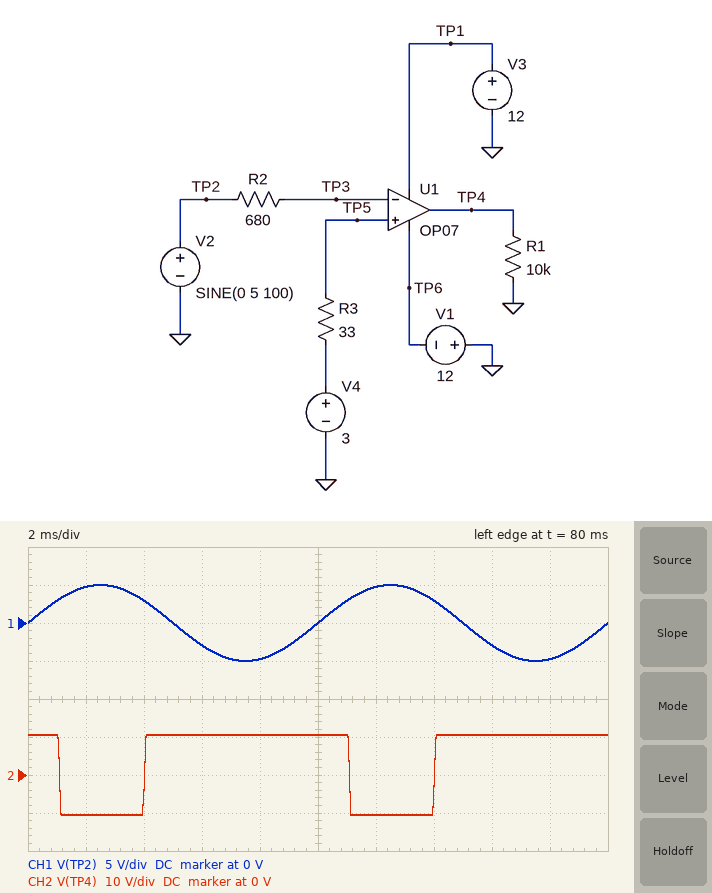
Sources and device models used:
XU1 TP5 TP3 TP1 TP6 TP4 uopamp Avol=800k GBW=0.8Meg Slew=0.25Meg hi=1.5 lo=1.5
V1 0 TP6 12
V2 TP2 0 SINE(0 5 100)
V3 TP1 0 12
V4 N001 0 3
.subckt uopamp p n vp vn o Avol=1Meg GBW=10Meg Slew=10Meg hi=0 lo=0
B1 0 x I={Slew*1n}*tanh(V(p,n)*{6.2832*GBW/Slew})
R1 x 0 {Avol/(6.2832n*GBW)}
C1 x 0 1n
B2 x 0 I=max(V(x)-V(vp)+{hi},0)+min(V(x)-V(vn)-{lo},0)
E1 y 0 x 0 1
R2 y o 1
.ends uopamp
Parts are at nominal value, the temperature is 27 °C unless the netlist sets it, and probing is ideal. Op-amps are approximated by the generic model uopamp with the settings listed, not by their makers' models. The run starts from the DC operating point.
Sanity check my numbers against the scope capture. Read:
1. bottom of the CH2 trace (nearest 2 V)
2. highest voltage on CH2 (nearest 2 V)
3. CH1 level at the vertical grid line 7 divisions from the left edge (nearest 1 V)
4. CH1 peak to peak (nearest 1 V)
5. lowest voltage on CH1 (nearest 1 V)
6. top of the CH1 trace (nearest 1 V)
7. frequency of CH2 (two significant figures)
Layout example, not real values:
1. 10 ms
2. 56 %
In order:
1. -10 V
2. 10 V
3. 3 V
4. 10 V
5. -5 V
6. 5 V
7. 100 Hz
